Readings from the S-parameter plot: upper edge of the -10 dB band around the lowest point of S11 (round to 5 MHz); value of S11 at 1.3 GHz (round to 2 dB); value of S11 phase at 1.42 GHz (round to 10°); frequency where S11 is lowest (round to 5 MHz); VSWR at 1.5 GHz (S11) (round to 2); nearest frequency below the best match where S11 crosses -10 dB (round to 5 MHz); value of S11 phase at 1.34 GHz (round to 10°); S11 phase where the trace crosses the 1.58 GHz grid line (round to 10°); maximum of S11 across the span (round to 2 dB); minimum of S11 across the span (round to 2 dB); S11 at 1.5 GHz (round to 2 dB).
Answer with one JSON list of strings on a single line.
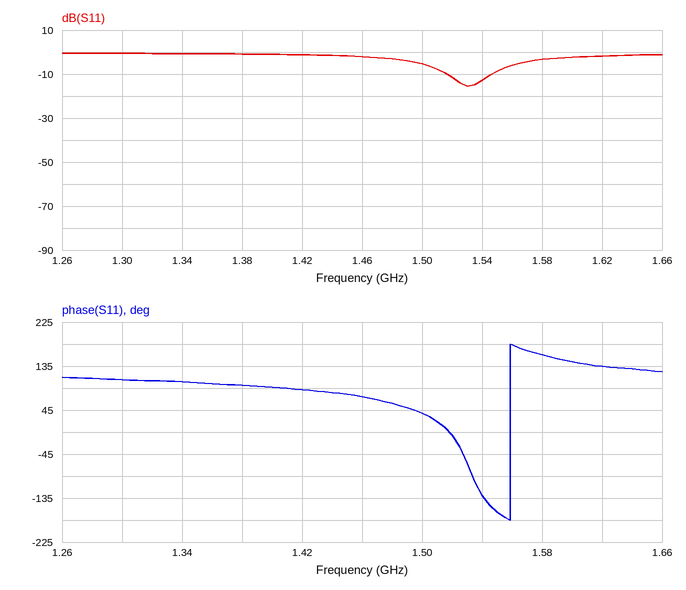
["1.545 GHz", "0 dB", "90°", "1.530 GHz", "4", "1.515 GHz", "100°", "160°", "0 dB", "-16 dB", "-6 dB"]
